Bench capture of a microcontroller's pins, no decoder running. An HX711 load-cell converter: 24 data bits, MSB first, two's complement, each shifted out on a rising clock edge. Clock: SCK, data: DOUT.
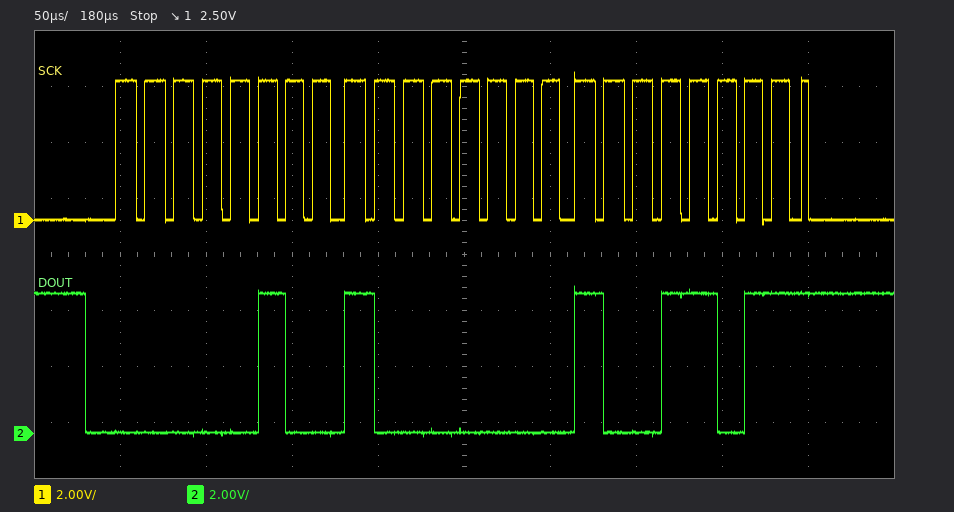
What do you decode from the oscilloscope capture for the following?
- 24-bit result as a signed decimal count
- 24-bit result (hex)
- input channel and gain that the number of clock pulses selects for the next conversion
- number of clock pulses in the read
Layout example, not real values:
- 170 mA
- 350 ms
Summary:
- 295067
- 0x04809B
- channel A, gain 128
- 25
